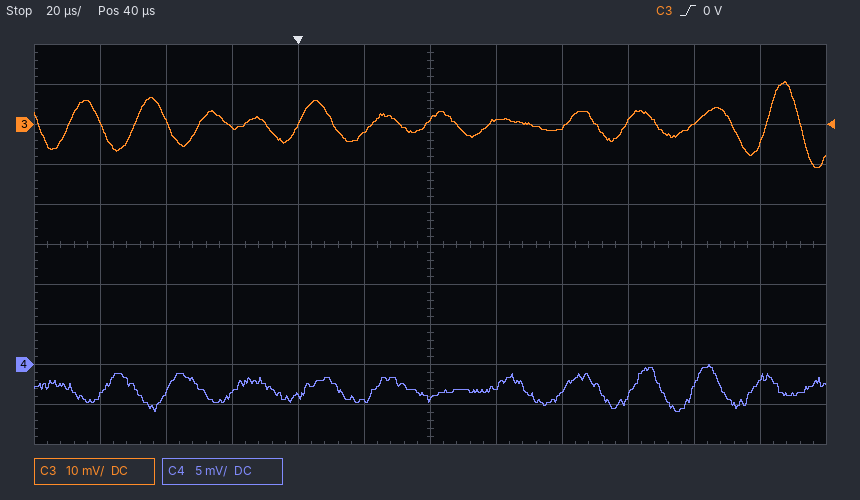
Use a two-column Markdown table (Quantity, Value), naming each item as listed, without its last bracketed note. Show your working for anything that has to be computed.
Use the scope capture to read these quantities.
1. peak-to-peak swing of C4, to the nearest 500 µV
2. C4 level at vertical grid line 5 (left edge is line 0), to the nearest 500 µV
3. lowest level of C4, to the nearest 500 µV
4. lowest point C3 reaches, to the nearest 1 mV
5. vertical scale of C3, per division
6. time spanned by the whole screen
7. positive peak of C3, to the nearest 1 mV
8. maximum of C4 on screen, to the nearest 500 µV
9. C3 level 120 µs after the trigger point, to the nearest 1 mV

| Quantity | Value |
|---|---|
| peak-to-peak swing of C4, to the nearest 500 µV | 0.0 mV − (-6.0 mV) = 6.0 mV |
| C4 level at vertical grid line 5 (left edge is line 0), to the nearest 500 µV | -4.5 mV |
| lowest level of C4, to the nearest 500 µV | -6.0 mV |
| lowest point C3 reaches, to the nearest 1 mV | -11 mV |
| vertical scale of C3, per division | 10 mV |
| time spanned by the whole screen | 240 µs |
| positive peak of C3, to the nearest 1 mV | 11 mV |
| maximum of C4 on screen, to the nearest 500 µV | 0.0 mV |
| C3 level 120 µs after the trigger point, to the nearest 1 mV | 0 mV |
